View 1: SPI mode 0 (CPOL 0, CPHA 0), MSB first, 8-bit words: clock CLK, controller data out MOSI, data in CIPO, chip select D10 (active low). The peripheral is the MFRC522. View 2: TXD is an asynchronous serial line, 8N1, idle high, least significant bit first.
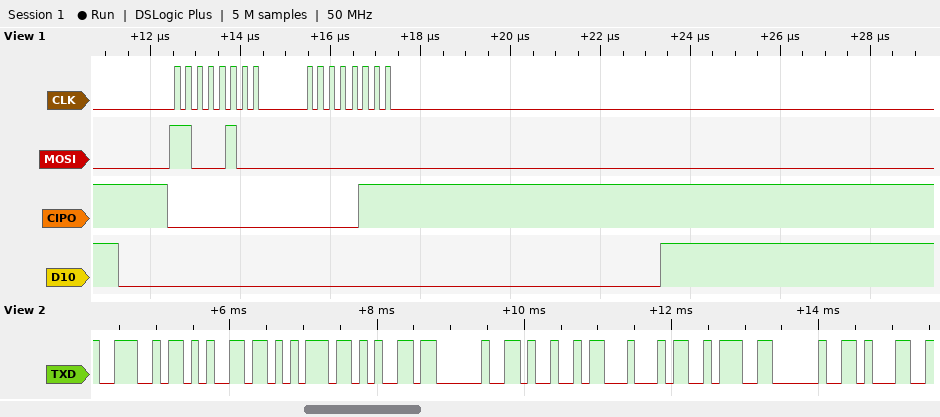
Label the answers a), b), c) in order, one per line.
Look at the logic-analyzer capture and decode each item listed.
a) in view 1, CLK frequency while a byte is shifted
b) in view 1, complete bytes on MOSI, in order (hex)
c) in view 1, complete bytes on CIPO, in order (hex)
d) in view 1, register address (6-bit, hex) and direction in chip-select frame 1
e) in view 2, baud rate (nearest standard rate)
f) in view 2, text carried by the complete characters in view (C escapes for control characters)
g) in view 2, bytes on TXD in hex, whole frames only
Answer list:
a) 4 MHz
b) C4 00
c) 00 07
d) 0x22 read
e) 9600 baud
f) "Neue ID: 1"
g) 4E 65 75 65 20 49 44 3A 20 31
